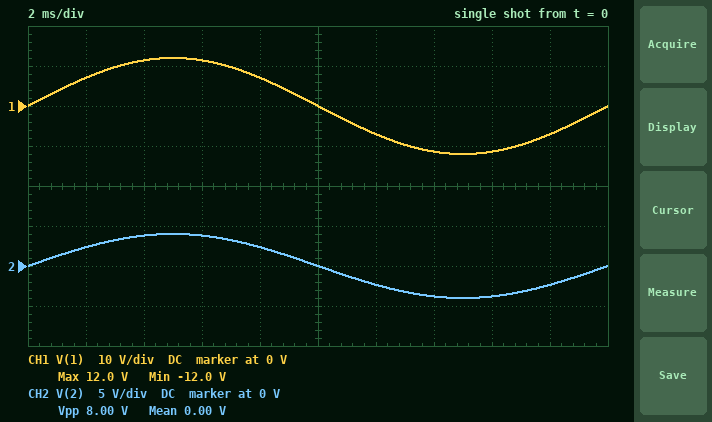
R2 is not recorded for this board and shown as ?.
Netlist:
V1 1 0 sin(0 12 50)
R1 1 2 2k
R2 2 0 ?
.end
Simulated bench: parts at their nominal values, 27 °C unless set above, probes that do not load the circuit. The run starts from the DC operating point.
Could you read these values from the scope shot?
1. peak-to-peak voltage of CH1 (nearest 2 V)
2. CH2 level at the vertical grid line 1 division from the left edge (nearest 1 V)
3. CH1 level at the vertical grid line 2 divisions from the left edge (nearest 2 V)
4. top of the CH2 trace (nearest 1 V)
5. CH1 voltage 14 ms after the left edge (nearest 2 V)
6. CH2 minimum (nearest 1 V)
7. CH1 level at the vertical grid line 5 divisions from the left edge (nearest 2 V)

24 V
2 V
12 V
4 V
-12 V
-4 V
0 V
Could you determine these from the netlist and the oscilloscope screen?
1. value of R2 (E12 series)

1 kΩ
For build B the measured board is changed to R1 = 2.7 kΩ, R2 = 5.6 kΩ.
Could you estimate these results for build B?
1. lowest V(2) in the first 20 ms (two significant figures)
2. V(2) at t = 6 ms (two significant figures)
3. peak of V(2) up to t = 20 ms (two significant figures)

-8.1 V
7.7 V
8.1 V
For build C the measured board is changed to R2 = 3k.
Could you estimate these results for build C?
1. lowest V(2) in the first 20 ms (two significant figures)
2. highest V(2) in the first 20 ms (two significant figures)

-7.2 V
7.2 V
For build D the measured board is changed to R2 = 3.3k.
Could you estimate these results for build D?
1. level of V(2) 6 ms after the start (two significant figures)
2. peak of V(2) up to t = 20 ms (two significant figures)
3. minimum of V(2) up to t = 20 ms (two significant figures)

7.1 V
7.5 V
-7.5 V
